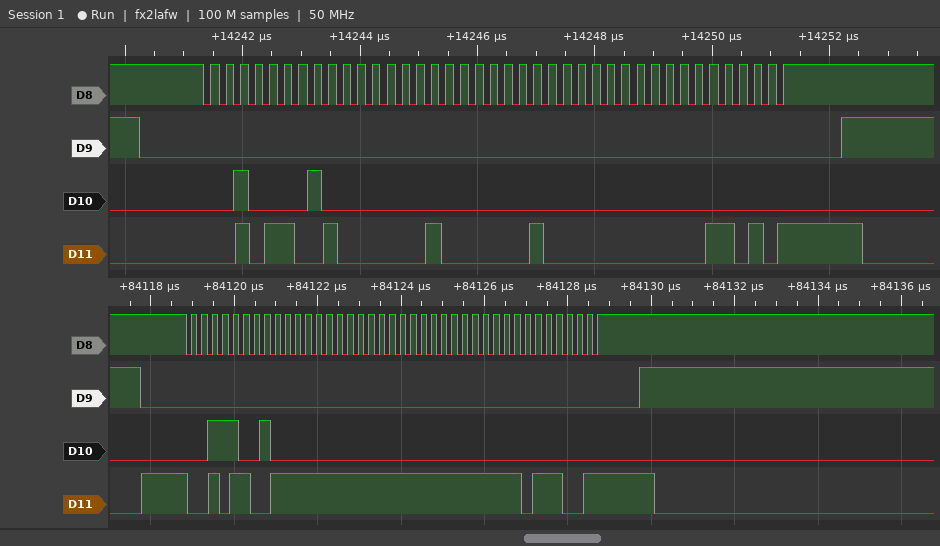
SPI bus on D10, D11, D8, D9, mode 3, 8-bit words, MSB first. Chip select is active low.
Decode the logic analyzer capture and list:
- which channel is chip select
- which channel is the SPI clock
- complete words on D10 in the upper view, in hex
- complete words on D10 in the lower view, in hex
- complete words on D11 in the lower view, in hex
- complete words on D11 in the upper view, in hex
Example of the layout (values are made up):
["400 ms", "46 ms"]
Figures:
["D9", "D8", "21, 00, 00, 00, 00", "39, 00, 00, 00, 00", "2C, FF, FF, FF, 73", "2C, 81, 02, 00, 35"]
